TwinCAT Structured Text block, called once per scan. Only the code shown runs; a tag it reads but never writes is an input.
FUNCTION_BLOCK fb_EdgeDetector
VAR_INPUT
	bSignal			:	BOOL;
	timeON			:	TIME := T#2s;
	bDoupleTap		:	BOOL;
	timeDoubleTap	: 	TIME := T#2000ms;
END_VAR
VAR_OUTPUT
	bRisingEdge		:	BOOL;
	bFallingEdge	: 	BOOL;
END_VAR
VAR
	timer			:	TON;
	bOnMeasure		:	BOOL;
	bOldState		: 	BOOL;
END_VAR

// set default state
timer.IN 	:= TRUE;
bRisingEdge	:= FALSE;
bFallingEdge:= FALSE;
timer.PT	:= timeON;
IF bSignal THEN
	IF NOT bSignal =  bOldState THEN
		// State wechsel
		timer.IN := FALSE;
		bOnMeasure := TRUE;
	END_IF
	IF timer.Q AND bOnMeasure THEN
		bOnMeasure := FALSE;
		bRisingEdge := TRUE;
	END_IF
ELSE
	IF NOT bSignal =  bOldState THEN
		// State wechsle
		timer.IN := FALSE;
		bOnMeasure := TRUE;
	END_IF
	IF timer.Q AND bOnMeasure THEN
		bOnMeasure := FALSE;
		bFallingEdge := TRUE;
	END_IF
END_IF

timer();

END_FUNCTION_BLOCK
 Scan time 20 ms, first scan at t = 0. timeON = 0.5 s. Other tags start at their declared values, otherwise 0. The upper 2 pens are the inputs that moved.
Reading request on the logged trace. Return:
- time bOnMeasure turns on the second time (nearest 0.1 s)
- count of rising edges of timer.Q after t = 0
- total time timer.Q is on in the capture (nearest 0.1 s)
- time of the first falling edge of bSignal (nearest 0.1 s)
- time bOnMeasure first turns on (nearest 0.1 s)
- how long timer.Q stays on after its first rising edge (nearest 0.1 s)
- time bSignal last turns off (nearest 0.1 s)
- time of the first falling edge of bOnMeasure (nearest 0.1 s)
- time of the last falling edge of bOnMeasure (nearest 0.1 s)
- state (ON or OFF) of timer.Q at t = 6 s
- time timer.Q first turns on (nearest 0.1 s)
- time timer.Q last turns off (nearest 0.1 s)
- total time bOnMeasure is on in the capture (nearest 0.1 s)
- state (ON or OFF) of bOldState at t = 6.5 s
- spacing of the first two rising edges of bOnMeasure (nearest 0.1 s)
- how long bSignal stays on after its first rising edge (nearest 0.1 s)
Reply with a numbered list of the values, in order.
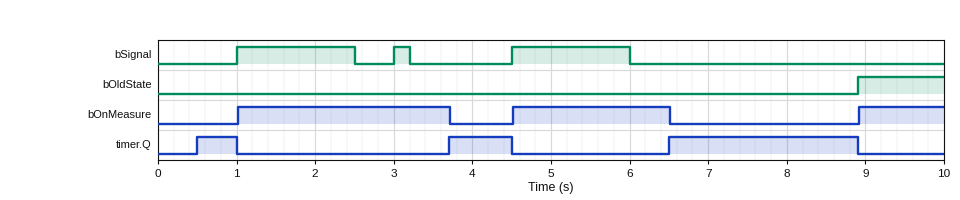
1. 4.5 s
2. 3
3. 3.7 s
4. 2.5 s
5. 1.0 s
6. 0.5 s
7. 6.0 s
8. 3.7 s
9. 6.5 s
10. OFF
11. 0.5 s
12. 8.9 s
13. 5.8 s
14. OFF
15. 3.5 s
16. 1.5 s
